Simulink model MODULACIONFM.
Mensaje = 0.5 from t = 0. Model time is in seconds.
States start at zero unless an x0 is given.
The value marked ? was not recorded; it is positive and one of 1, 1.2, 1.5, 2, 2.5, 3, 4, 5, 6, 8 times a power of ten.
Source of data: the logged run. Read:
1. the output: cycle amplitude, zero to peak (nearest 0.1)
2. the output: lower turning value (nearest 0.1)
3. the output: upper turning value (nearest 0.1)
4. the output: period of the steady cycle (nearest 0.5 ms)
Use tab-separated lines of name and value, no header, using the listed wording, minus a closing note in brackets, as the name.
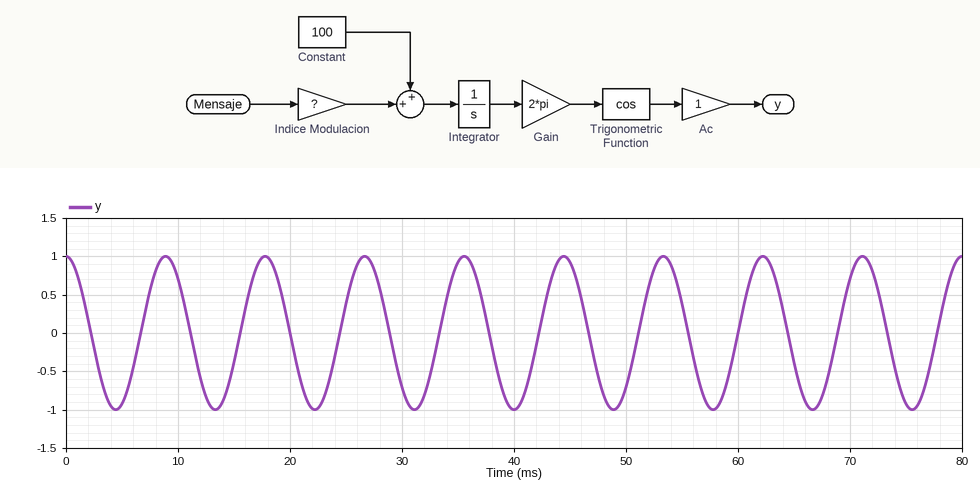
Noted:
the output: cycle amplitude, zero to peak	1.0
the output: lower turning value	-1.0
the output: upper turning value	1.0
the output: period of the steady cycle	9.0 ms
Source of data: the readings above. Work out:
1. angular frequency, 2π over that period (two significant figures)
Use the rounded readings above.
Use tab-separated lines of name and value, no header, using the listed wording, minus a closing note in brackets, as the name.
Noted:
angular frequency, 2π over that period	0.70 rad/ms
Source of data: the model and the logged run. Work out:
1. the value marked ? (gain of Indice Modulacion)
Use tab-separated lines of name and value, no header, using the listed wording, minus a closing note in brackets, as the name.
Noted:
the value marked ?	25
